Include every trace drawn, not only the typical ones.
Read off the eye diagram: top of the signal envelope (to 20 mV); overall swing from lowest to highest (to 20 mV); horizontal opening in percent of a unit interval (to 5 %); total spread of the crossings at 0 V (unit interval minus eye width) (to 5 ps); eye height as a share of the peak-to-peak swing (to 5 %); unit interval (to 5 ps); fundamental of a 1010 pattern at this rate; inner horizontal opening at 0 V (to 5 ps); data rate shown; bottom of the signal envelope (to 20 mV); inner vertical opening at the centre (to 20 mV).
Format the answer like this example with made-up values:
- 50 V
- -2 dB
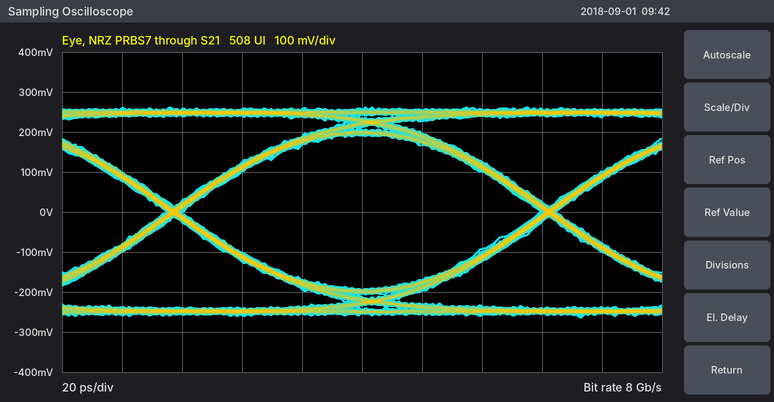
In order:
- 260 mV
- 520 mV
- 95 %
- 5 ps
- 75 %
- 125 ps
- 4 GHz
- 120 ps
- 8 Gb/s
- -260 mV
- 380 mV
